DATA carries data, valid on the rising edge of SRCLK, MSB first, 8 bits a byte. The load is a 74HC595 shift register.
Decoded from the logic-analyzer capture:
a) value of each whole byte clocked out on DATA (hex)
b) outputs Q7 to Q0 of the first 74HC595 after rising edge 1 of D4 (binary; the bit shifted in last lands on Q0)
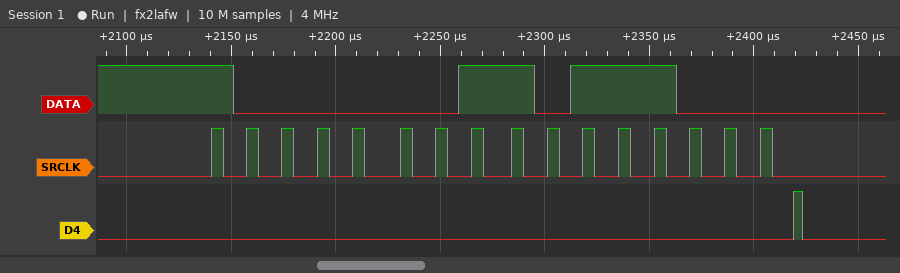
0x81 0xB8
10111000
